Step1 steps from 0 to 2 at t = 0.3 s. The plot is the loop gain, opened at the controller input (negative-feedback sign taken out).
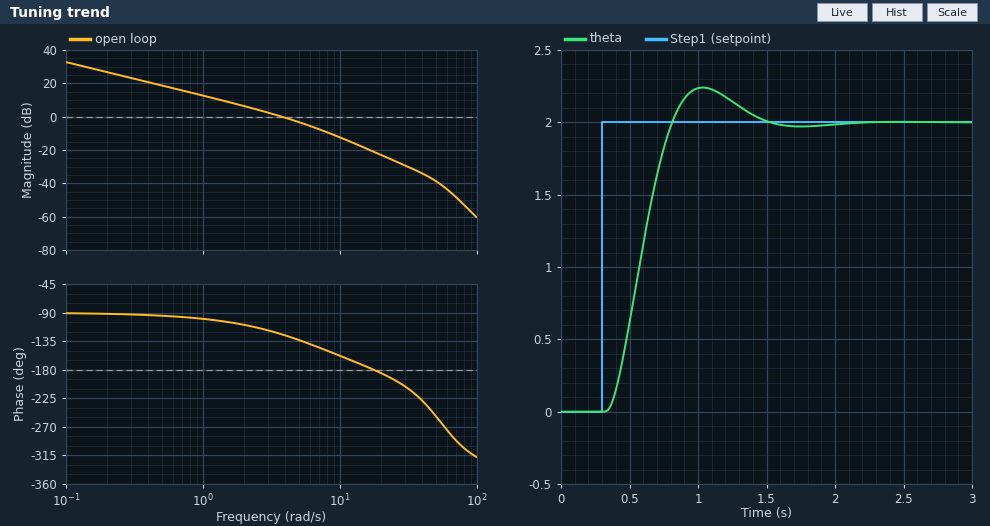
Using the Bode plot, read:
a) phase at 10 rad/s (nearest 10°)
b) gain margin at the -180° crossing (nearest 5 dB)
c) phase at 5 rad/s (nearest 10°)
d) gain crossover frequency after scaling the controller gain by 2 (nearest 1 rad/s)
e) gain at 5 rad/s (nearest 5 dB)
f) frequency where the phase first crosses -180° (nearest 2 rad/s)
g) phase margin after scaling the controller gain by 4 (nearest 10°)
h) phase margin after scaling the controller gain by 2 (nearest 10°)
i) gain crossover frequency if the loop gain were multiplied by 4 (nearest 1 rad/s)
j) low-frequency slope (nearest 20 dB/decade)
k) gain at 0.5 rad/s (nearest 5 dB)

-160°
20 dB
-130°
6 rad/s
-5 dB
18 rad/s
20°
40°
10 rad/s
-20 dB/decade
20 dB
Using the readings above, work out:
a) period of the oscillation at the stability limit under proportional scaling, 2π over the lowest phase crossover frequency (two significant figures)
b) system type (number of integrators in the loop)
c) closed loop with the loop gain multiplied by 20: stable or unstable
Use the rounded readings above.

0.35 s
1
unstable
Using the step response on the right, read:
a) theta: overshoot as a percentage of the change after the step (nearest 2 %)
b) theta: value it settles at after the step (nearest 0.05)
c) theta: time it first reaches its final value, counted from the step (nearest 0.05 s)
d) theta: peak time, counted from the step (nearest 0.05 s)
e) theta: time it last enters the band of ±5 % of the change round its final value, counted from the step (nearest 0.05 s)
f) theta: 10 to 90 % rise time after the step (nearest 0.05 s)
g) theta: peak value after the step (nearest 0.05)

12 %
2.00
0.50 s
0.75 s
1.00 s
0.35 s
2.25
